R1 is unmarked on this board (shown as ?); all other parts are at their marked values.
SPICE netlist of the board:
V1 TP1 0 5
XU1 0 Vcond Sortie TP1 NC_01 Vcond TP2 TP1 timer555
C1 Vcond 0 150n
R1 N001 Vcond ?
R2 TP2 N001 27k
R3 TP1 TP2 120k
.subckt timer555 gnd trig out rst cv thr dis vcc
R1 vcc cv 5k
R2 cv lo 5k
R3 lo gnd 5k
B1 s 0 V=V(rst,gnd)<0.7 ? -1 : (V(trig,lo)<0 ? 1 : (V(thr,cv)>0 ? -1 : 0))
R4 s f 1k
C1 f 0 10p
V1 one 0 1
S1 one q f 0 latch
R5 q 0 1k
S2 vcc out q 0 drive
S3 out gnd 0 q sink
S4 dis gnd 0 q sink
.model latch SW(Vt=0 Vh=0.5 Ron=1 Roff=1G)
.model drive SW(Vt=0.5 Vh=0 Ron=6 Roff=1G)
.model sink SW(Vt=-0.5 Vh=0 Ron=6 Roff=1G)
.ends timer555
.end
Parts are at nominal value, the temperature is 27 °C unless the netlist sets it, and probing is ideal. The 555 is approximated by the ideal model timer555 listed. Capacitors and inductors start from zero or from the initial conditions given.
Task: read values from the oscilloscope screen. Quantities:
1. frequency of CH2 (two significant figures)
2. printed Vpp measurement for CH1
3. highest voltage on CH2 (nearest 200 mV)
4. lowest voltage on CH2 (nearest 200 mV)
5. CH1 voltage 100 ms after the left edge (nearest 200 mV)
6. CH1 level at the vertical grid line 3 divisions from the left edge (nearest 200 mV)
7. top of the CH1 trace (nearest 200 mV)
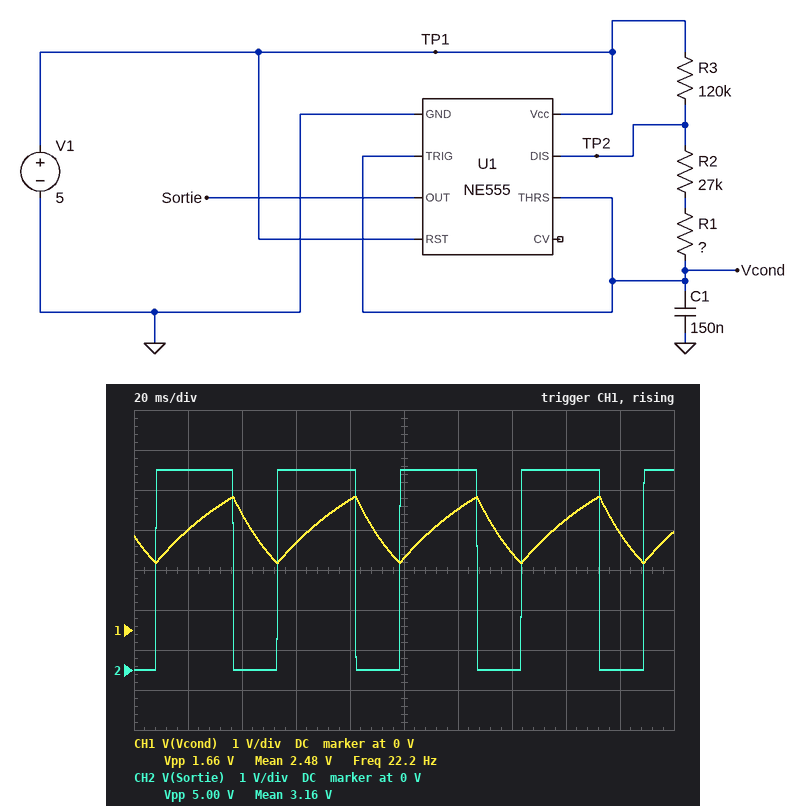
22 Hz
1.66 V
5.0 V
0 V
1.8 V
2.2 V
3.4 V
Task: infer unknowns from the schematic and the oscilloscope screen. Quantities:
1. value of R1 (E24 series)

130 kΩ
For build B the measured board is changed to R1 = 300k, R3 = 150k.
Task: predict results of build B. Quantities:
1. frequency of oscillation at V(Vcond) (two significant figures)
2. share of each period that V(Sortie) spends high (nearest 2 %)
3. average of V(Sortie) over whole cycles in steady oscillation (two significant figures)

12 Hz
60 %
3.0 V
